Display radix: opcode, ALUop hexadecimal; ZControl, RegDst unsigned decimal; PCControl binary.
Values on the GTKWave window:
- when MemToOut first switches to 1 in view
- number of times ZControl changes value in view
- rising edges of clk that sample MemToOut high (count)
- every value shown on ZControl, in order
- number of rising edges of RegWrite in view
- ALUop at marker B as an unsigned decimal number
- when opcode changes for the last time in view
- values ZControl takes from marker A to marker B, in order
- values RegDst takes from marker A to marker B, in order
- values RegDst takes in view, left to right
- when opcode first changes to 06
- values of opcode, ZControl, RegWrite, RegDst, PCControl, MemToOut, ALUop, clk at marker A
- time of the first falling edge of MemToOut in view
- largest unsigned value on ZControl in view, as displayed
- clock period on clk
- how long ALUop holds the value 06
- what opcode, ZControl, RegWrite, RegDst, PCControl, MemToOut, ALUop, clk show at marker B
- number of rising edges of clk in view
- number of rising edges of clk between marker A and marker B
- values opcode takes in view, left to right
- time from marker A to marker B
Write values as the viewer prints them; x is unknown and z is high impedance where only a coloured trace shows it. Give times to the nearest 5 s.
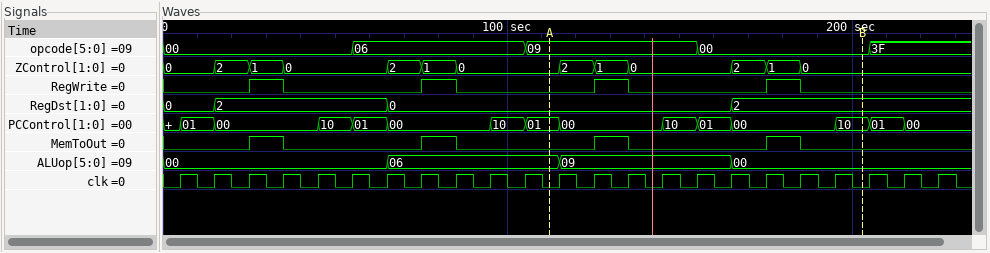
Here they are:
25 s
12
4
0, 2, 1, 0, 2, 1, 0, 2, 1, 0, 2, 1, 0
4
0
205 s
0, 2, 1, 0, 2, 1, 0
0, 2
0, 2, 0, 2
55 s
opcode=09, ZControl=0, RegWrite=0, RegDst=0, PCControl=01, MemToOut=0, ALUop=06, clk=0
35 s
2
10 s
50 s
opcode=00, ZControl=0, RegWrite=0, RegDst=2, PCControl=10, MemToOut=0, ALUop=00, clk=0
23
9
00, 06, 09, 00, 3F
90 s
